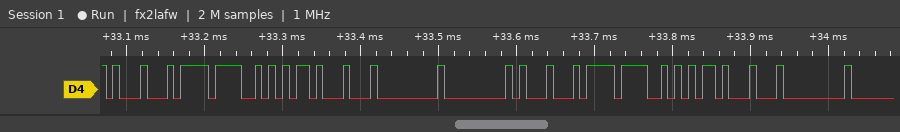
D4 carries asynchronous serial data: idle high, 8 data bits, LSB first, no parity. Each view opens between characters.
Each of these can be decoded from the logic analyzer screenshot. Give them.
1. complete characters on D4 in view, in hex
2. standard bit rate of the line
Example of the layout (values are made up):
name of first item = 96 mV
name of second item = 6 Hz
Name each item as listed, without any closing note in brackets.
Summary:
complete characters on D4 in view, in hex = 11, EF, AA, 11, 00, 00, 11, EF, AA, 11, 00
standard bit rate of the line = 115200 baud
